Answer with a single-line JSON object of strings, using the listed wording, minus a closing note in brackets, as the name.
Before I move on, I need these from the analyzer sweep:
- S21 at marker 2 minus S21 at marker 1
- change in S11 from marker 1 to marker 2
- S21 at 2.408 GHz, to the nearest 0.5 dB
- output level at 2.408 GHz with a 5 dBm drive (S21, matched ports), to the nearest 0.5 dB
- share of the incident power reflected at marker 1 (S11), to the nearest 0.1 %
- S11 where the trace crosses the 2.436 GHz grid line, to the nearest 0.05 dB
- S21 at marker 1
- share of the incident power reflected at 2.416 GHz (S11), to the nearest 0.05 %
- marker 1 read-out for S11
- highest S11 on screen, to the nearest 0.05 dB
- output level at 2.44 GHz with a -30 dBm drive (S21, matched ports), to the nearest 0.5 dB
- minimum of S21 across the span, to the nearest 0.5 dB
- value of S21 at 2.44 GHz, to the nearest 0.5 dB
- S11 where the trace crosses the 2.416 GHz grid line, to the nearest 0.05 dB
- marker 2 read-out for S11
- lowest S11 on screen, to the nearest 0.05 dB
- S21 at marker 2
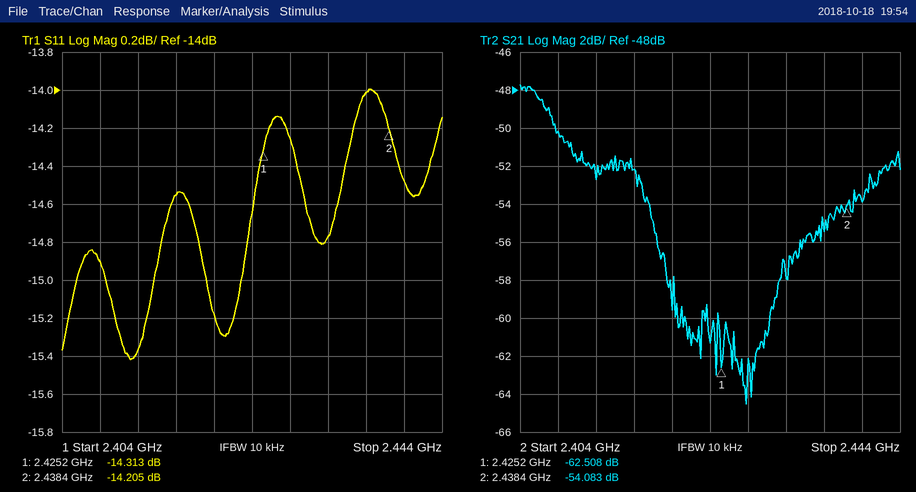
{"S21 at marker 2 minus S21 at marker 1": "8.425 dB", "change in S11 from marker 1 to marker 2": "0.108 dB", "S21 at 2.408 GHz, to the nearest 0.5 dB": "-50.0 dB", "output level at 2.408 GHz with a 5 dBm drive (S21, matched ports), to the nearest 0.5 dB": "-45.0 dBm", "share of the incident power reflected at marker 1 (S11), to the nearest 0.1 %": "3.7 %", "S11 where the trace crosses the 2.436 GHz grid line, to the nearest 0.05 dB": "-14.00 dB", "S21 at marker 1": "-62.508 dB", "share of the incident power reflected at 2.416 GHz (S11), to the nearest 0.05 %": "3.50 %", "marker 1 read-out for S11": "-14.313 dB", "highest S11 on screen, to the nearest 0.05 dB": "-14.00 dB", "output level at 2.44 GHz with a -30 dBm drive (S21, matched ports), to the nearest 0.5 dB": "-84.0 dBm", "minimum of S21 across the span, to the nearest 0.5 dB": "-64.5 dB", "value of S21 at 2.44 GHz, to the nearest 0.5 dB": "-54.0 dB", "S11 where the trace crosses the 2.416 GHz grid line, to the nearest 0.05 dB": "-14.55 dB", "marker 2 read-out for S11": "-14.205 dB", "lowest S11 on screen, to the nearest 0.05 dB": "-15.40 dB", "S21 at marker 2": "-54.083 dB"}
